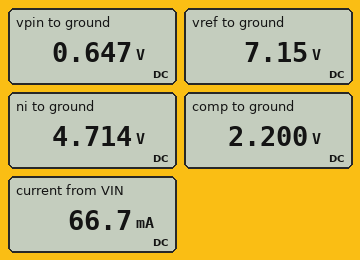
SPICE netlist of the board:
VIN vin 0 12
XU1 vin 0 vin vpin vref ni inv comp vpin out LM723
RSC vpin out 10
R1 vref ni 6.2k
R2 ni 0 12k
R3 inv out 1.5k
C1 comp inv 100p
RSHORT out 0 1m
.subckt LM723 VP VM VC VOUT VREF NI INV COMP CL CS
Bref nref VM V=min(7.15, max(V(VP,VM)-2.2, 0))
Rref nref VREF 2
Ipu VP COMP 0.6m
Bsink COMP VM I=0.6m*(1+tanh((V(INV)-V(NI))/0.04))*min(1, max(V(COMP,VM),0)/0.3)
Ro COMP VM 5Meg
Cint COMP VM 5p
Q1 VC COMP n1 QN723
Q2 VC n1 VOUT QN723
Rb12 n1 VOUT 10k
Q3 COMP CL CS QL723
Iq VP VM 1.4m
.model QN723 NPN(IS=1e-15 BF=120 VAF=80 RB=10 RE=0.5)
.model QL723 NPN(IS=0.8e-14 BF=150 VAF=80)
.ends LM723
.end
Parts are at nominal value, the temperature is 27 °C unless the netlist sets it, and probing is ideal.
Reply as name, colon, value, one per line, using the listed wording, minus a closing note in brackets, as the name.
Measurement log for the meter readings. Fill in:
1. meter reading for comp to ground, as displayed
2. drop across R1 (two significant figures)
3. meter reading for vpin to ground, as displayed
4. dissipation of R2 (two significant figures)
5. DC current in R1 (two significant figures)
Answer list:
meter reading for comp to ground, as displayed: 2.200 V
drop across R1: 2.4 V
meter reading for vpin to ground, as displayed: 0.647 V
dissipation of R2: 1.9 mW
DC current in R1: 390 µA
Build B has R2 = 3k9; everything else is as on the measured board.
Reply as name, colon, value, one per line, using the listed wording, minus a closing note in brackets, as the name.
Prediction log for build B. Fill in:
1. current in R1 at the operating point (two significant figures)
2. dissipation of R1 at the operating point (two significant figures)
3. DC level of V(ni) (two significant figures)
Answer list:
current in R1 at the operating point: 710 µA
dissipation of R1 at the operating point: 3.1 mW
DC level of V(ni): 2.8 V
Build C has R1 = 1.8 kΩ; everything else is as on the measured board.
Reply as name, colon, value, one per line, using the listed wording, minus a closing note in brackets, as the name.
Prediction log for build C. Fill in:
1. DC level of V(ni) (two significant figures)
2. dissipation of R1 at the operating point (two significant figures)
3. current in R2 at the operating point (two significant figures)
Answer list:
DC level of V(ni): 6.2 V
dissipation of R1 at the operating point: 480 µW
current in R2 at the operating point: 520 µA
